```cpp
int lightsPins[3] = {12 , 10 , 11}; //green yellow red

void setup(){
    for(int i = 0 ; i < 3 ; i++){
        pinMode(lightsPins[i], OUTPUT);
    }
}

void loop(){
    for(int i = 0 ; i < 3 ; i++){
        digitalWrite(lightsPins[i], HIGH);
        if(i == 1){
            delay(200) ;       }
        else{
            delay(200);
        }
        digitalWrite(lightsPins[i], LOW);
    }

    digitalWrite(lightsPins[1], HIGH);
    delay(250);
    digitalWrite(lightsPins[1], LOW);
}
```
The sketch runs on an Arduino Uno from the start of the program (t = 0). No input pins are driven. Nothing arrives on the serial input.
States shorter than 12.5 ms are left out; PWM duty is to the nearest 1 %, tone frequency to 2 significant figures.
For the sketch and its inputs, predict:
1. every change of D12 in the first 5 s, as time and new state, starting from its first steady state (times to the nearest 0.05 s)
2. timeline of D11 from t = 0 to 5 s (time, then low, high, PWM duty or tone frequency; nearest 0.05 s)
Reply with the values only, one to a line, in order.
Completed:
0 s high; 0.2 s low; 0.85 s high; 1.05 s low; 1.7 s high; 1.9 s low; 2.55 s high; 2.75 s low; 3.4 s high; 3.6 s low; 4.25 s high; 4.45 s low
0 s low; 0.4 s high; 0.6 s low; 1.25 s high; 1.45 s low; 2.1 s high; 2.3 s low; 2.95 s high; 3.15 s low; 3.8 s high; 4 s low; 4.65 s high; 4.85 s low
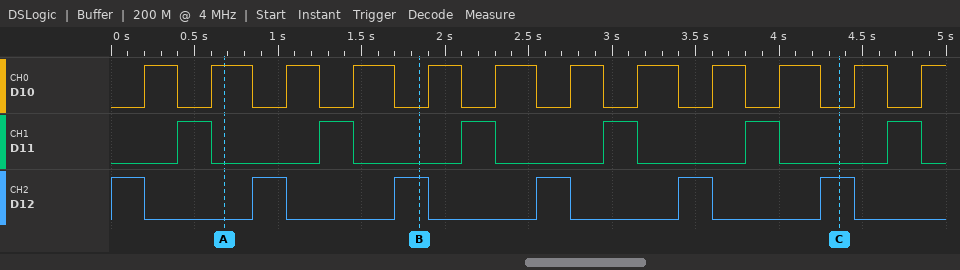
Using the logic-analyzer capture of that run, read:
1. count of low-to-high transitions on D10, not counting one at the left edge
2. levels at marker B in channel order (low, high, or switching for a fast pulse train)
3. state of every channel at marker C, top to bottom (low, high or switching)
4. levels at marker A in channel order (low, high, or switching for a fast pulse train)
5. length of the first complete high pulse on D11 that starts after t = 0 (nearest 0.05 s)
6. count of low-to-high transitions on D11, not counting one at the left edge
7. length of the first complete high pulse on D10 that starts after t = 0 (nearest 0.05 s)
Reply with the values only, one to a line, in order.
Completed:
12
D10 low, D11 low, D12 high
D10 low, D11 low, D12 high
D10 high, D11 low, D12 low
0.20 s
6
0.20 s
